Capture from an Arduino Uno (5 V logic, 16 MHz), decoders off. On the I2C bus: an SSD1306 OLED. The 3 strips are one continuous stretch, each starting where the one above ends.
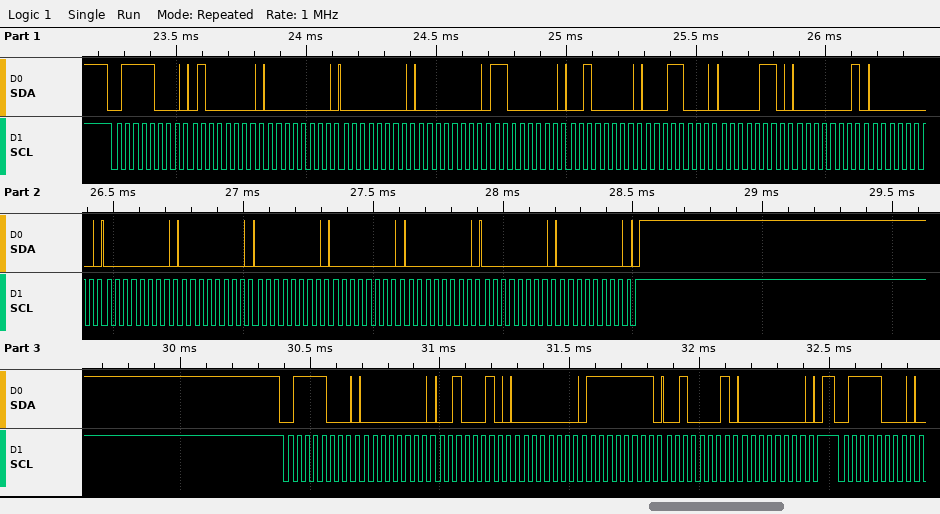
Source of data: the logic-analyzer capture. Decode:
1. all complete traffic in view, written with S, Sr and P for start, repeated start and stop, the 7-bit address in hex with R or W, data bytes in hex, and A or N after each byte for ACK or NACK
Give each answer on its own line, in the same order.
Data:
S 3CW A 40 A 00 A 00 A 00 A C0 A 20 A 18 A 06 A 01 A 00 A 00 A 00 A 00 A 00 A 00 A 00 A 00 A P S 3CW A 00 A 22 A 00 A FF A 21 A 00 A P S 3CW A
